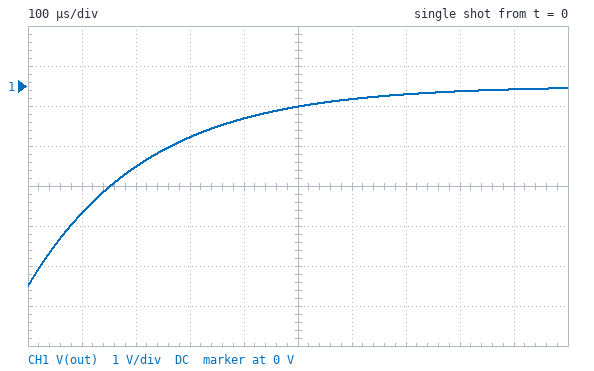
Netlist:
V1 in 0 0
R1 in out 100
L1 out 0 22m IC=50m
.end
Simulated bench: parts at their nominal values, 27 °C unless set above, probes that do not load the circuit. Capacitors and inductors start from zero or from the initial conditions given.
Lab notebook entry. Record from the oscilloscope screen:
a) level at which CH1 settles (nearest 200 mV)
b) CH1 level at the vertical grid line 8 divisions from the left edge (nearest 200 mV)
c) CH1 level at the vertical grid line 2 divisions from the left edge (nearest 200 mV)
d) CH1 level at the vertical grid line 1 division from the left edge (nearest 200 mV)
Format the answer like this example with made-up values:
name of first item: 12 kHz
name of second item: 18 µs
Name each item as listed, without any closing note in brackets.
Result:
level at which CH1 settles: 0 V
CH1 level at the vertical grid line 8 divisions from the left edge: -200 mV
CH1 level at the vertical grid line 2 divisions from the left edge: -2.0 V
CH1 level at the vertical grid line 1 division from the left edge: -3.2 V
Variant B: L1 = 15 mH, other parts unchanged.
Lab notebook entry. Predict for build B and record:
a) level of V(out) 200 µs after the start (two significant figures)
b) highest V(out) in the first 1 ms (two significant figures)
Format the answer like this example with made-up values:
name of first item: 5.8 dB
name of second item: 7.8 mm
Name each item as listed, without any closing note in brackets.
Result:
level of V(out) 200 µs after the start: -1.3 V
highest V(out) in the first 1 ms: -6.4 mV
